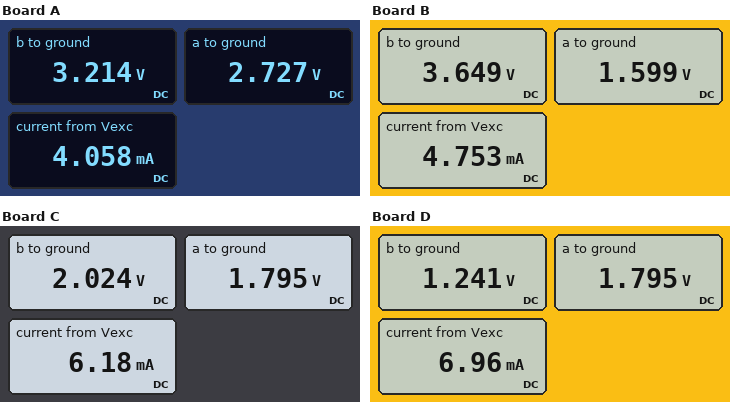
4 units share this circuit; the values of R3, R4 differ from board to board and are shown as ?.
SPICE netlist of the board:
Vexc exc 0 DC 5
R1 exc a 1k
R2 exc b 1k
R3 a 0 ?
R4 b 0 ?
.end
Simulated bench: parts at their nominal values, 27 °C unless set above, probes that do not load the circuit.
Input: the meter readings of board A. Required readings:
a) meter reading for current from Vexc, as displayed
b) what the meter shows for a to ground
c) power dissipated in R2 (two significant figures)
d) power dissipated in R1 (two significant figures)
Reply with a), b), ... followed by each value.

a) 4.058 mA
b) 2.727 V
c) 3.2 mW
d) 5.2 mW
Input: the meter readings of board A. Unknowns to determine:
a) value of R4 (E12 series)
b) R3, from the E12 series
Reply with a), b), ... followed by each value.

a) 1.8 kΩ
b) 1.2 kΩ
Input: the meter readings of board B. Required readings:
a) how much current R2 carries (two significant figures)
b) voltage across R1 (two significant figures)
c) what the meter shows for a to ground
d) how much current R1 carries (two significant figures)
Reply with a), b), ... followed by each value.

a) 1.4 mA
b) 3.4 V
c) 1.599 V
d) 3.4 mA
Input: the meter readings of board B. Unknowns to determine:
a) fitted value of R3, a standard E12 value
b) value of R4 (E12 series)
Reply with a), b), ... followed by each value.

a) 470 Ω
b) 2.7 kΩ
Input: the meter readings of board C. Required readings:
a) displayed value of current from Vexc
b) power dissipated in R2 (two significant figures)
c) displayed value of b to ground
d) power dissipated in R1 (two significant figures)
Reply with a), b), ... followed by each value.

a) 6.18 mA
b) 8.9 mW
c) 2.024 V
d) 10 mW
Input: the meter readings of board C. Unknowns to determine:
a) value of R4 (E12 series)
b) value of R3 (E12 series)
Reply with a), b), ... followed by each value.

a) 680 Ω
b) 560 Ω
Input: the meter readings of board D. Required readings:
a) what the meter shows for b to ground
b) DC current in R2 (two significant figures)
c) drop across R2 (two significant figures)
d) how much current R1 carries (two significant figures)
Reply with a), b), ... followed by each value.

a) 1.241 V
b) 3.8 mA
c) 3.8 V
d) 3.2 mA
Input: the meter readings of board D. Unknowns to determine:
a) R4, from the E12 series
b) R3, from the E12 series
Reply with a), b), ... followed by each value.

a) 330 Ω
b) 560 Ω
